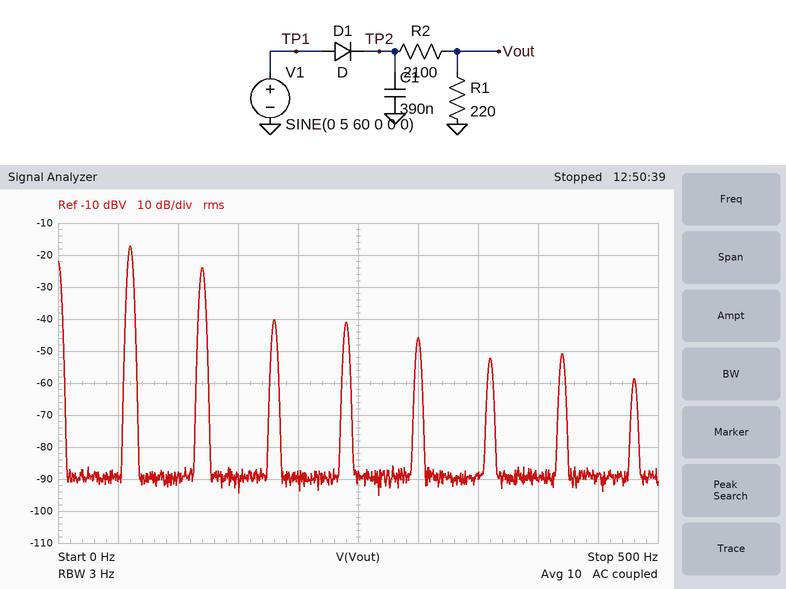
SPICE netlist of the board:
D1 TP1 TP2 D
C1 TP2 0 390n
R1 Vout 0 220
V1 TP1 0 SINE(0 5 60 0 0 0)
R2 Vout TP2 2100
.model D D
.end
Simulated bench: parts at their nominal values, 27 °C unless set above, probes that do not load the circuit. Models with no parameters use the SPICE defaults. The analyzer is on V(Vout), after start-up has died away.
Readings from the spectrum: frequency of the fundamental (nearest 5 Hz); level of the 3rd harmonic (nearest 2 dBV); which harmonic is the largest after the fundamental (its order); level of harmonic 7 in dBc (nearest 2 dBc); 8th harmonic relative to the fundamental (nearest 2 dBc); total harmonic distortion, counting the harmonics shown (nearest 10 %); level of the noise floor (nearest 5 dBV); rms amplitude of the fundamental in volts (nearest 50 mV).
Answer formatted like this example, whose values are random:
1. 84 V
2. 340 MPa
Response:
1. 60 Hz
2. -40 dBV
3. 2
4. -34 dBc
5. -42 dBc
6. 50 %
7. -90 dBV
8. 150 mV
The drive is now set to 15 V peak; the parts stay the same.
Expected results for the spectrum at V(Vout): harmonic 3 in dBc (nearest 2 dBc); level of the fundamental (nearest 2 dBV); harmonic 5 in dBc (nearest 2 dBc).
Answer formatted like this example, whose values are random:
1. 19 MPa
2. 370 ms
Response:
1. -28 dBc
2. -6 dBV
3. -32 dBc
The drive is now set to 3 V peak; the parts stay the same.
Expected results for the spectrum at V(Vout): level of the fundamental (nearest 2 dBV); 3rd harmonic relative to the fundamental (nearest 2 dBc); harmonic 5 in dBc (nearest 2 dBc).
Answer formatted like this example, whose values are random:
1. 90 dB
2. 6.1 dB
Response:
1. -22 dBV
2. -20 dBc
3. -26 dBc
